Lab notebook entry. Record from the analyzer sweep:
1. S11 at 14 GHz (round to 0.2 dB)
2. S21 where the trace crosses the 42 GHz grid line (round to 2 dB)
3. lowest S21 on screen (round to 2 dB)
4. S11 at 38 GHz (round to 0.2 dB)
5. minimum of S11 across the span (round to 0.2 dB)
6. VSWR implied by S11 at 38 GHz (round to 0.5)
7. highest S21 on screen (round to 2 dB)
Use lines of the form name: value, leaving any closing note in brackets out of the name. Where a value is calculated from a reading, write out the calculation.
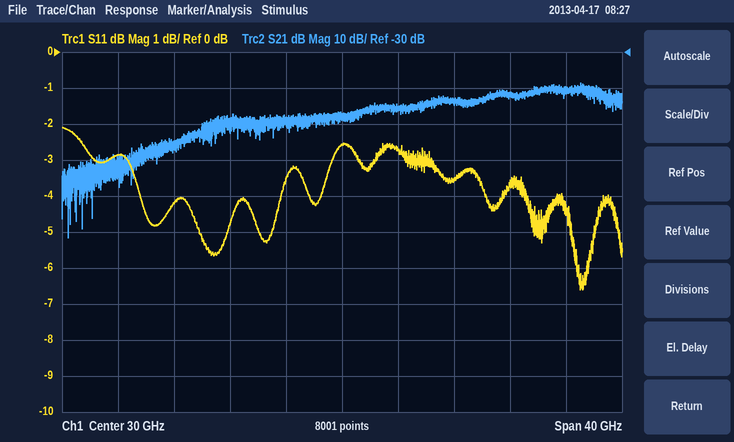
S11 at 14 GHz: -2.8 dB
S21 where the trace crosses the 42 GHz grid line: -42 dB
lowest S21 on screen: -82 dB
S11 at 38 GHz: -3.6 dB
minimum of S11 across the span: -6.6 dB
VSWR implied by S11 at 38 GHz: |Γ| = 10^(-3.6/20) = 0.6607; VSWR = (1 + 0.6607)/(1 − 0.6607) ≈ 4.89, so 5.0 to the nearest 0.5
highest S21 on screen: -38 dB
